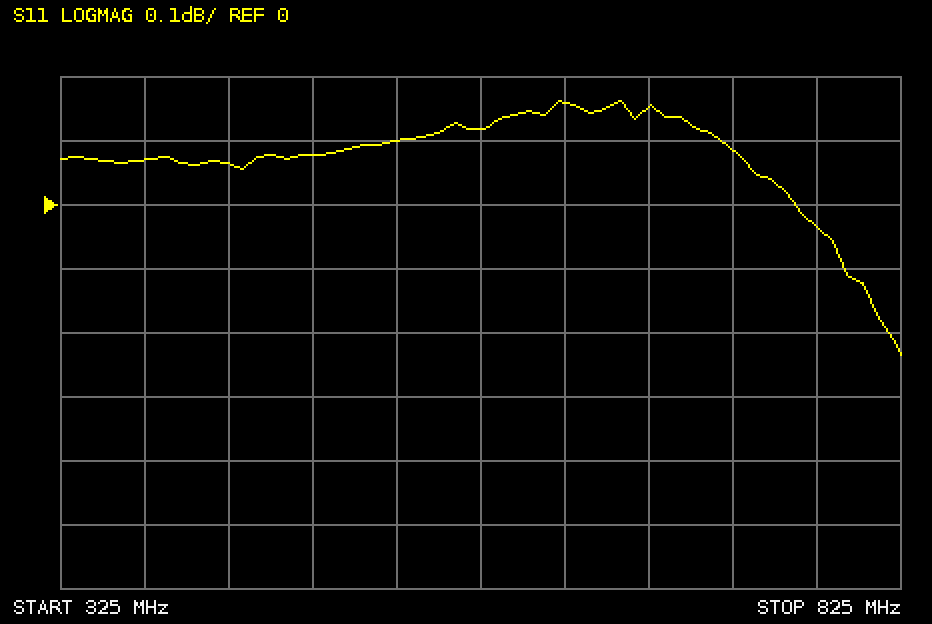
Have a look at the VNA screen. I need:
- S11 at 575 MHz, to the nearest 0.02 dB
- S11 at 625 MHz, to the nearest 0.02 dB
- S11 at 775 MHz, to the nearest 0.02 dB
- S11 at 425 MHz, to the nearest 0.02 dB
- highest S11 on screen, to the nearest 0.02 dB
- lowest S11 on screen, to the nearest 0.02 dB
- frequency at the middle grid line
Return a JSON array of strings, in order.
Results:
["0.12 dB", "0.16 dB", "-0.04 dB", "0.06 dB", "0.16 dB", "-0.24 dB", "575 MHz"]
